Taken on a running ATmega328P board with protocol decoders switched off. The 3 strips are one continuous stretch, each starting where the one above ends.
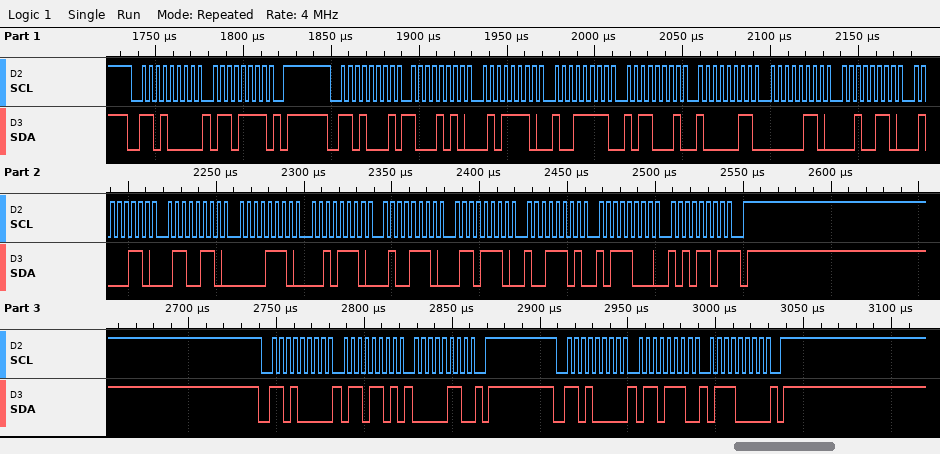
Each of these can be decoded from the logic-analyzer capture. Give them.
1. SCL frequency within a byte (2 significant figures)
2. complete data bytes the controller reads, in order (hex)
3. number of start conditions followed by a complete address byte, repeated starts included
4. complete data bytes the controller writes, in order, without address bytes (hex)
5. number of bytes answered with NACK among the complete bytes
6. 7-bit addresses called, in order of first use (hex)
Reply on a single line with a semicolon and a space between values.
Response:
250 kHz; 8A 5E 9F B1 83 06 26 46 66 0E 2E 4E 6E 9D B8 AD; 4; 6F 6D 06 6E 70; 1; 0x68
